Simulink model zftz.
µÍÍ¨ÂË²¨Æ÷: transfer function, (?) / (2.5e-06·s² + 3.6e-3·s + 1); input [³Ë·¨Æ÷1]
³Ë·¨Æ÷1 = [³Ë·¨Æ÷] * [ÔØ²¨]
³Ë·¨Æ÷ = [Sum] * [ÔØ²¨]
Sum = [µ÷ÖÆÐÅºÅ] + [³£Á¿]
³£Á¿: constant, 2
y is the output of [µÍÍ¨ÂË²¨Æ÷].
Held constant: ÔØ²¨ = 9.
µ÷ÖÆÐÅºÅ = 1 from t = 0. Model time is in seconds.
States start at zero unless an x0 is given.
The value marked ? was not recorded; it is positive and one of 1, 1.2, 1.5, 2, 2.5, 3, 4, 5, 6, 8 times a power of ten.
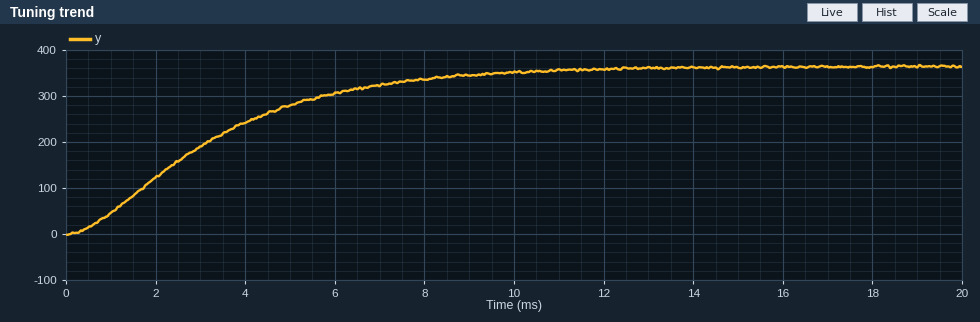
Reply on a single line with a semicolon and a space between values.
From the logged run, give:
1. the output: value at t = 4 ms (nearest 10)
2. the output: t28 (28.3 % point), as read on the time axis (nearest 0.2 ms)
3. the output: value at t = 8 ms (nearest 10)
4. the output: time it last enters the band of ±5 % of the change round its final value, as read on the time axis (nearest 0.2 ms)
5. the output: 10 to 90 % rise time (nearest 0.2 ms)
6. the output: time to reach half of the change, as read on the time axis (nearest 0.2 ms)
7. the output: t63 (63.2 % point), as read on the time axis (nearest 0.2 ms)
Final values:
240; 1.8 ms; 340; 9.2 ms; 6.4 ms; 2.8 ms; 3.8 ms
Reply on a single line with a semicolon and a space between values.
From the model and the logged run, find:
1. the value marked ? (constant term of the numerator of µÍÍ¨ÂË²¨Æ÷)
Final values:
1.5
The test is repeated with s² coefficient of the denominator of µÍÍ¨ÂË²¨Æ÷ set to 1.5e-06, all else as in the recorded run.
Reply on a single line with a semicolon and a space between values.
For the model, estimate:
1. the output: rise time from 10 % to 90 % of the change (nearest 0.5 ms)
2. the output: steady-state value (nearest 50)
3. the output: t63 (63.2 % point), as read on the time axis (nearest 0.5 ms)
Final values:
7.0 ms; 350; 3.5 ms
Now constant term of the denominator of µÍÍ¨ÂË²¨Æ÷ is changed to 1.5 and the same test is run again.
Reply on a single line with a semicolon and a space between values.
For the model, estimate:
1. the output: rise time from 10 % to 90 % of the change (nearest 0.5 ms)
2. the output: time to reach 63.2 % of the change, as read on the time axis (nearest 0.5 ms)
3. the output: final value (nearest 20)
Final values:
4.0 ms; 2.5 ms; 240
